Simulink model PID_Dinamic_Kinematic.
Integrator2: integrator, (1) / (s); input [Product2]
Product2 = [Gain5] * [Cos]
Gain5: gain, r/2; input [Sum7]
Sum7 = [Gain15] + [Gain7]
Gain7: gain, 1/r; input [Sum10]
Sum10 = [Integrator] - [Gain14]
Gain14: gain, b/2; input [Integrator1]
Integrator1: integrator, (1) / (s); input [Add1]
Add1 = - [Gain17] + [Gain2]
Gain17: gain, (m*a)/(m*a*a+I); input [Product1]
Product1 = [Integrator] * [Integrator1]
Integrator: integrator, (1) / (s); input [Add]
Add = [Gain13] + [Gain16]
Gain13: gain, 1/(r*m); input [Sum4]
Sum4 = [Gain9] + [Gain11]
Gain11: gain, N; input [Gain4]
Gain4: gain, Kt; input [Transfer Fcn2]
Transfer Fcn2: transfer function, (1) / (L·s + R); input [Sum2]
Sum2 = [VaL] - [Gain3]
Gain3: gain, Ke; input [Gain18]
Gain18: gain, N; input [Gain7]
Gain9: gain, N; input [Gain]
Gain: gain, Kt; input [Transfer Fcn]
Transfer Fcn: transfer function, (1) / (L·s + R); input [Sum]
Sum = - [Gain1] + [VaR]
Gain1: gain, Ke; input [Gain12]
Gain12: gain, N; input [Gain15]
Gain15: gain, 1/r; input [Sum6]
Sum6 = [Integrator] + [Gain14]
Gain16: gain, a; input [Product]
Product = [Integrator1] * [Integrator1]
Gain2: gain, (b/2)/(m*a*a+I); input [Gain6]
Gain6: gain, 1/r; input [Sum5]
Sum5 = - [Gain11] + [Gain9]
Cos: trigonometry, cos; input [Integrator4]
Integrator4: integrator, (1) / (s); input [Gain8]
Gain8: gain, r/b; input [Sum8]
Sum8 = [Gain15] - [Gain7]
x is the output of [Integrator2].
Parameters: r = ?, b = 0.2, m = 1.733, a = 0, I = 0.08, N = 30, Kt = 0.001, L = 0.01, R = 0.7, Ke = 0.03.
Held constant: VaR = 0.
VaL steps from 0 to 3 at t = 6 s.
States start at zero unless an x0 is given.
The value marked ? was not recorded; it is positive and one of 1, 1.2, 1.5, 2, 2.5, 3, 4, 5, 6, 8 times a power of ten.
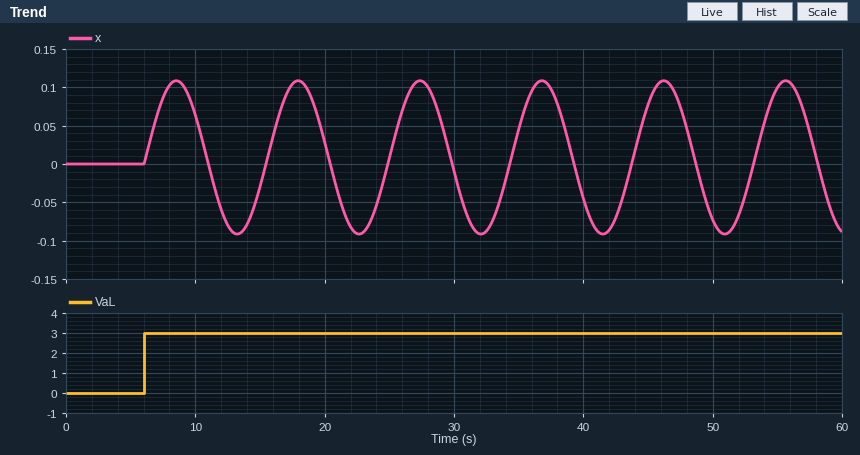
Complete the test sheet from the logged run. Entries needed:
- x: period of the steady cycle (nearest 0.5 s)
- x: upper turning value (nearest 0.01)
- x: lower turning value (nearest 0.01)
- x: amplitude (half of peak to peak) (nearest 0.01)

9.5 s
0.11
-0.09
0.10
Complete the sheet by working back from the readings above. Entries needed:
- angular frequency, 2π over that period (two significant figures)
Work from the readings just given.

0.66 rad/s
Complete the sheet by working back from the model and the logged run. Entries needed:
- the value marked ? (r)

0.04
